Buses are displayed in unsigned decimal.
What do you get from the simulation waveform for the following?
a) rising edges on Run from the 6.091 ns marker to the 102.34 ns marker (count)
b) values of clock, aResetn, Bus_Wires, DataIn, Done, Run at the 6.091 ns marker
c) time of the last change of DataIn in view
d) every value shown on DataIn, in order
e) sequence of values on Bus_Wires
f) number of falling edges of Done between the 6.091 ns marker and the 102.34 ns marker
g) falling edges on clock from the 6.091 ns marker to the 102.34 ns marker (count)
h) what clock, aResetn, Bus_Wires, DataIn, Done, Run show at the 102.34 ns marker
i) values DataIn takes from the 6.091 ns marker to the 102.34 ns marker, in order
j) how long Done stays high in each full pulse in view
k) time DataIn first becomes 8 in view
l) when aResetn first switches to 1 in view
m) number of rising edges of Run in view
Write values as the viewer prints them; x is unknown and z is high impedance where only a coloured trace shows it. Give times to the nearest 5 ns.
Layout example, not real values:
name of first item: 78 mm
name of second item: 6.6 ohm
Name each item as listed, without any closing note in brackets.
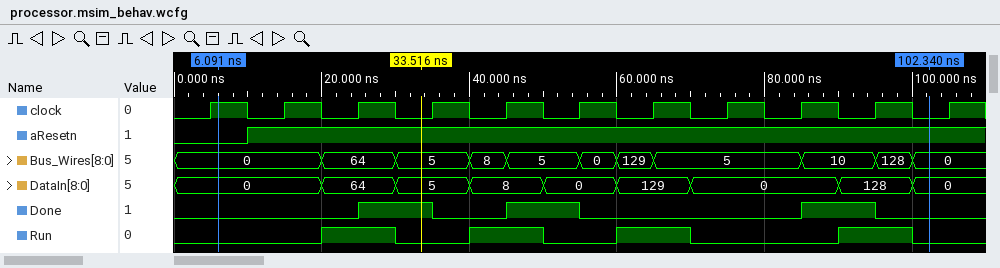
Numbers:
rising edges on Run from the 6.091 ns marker to the 102.34 ns marker: 4
values of clock, aResetn, Bus_Wires, DataIn, Done, Run at the 6.091 ns marker: clock=1, aResetn=0, Bus_Wires=0, DataIn=0, Done=0, Run=0
time of the last change of DataIn in view: 100 ns
every value shown on DataIn, in order: 0, 64, 5, 8, 0, 129, 0, 128, 0
sequence of values on Bus_Wires: 0, 64, 5, 8, 5, 0, 129, 5, 10, 128, 0
number of falling edges of Done between the 6.091 ns marker and the 102.34 ns marker: 3
falling edges on clock from the 6.091 ns marker to the 102.34 ns marker: 10
what clock, aResetn, Bus_Wires, DataIn, Done, Run show at the 102.34 ns marker: clock=0, aResetn=1, Bus_Wires=0, DataIn=0, Done=0, Run=0
values DataIn takes from the 6.091 ns marker to the 102.34 ns marker, in order: 0, 64, 5, 8, 0, 129, 0, 128, 0
how long Done stays high in each full pulse in view: 10 ns, 10 ns, 10 ns
time DataIn first becomes 8 in view: 40 ns
when aResetn first switches to 1 in view: 10 ns
number of rising edges of Run in view: 4
